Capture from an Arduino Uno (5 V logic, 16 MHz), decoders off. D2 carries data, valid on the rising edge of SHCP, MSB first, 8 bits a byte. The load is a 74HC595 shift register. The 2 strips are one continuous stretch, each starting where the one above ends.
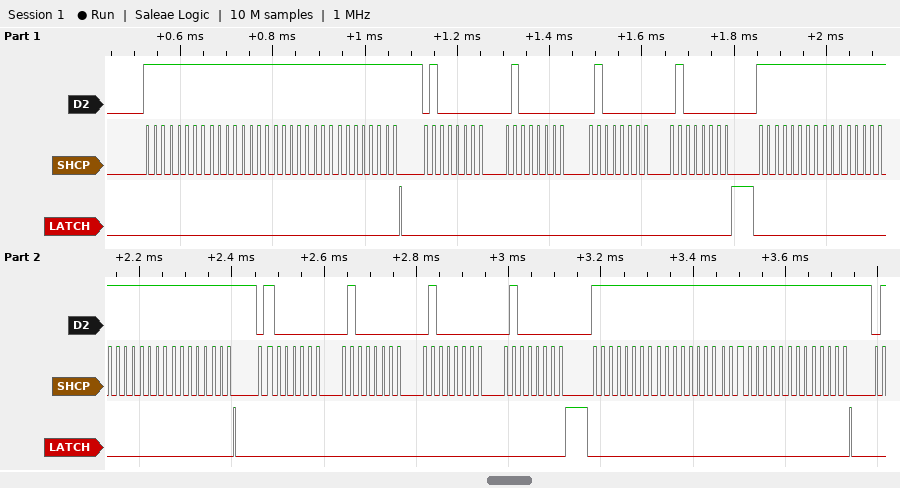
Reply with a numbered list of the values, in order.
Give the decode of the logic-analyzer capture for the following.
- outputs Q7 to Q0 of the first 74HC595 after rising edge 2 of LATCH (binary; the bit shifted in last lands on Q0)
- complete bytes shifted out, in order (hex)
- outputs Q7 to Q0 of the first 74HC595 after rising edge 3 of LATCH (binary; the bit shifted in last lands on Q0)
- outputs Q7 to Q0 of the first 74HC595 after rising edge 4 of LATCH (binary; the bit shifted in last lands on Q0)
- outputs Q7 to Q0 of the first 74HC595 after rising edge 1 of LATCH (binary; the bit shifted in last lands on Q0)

1. 01000000
2. 0xFF 0xFF 0xFF 0xFF 0x40 0x40 0x40 0x40 0xFF 0xFF 0xFF 0xFF 0x40 0x40 0x40 0x40 0xFF 0xFF 0xFF 0xFF
3. 11111111
4. 01000000
5. 11111111
